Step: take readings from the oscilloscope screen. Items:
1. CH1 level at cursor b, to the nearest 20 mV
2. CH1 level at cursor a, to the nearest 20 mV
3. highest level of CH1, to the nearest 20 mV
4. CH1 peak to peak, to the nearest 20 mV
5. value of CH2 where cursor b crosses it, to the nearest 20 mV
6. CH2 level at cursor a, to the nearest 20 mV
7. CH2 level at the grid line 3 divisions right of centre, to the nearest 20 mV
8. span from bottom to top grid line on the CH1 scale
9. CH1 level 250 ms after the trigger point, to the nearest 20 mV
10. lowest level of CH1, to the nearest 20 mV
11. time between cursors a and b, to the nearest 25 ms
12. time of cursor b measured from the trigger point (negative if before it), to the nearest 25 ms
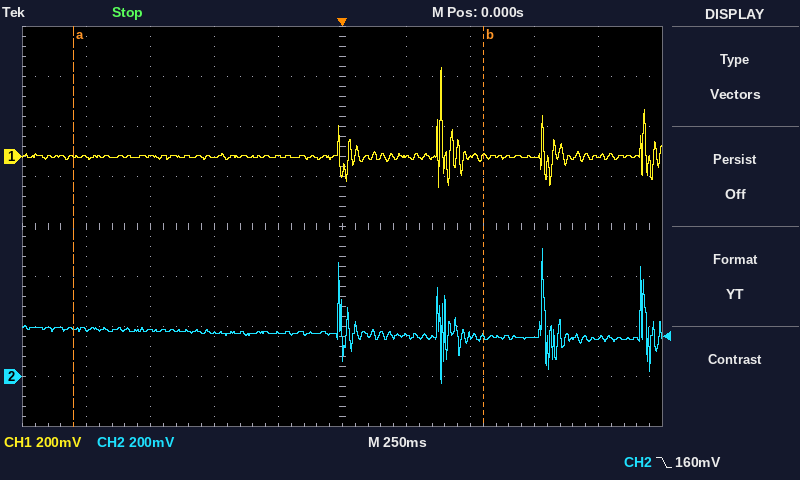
0 mV
0 mV
360 mV
480 mV
160 mV
200 mV
160 mV
1.6 V
0 mV
-120 mV
1.600 s
+550 ms
